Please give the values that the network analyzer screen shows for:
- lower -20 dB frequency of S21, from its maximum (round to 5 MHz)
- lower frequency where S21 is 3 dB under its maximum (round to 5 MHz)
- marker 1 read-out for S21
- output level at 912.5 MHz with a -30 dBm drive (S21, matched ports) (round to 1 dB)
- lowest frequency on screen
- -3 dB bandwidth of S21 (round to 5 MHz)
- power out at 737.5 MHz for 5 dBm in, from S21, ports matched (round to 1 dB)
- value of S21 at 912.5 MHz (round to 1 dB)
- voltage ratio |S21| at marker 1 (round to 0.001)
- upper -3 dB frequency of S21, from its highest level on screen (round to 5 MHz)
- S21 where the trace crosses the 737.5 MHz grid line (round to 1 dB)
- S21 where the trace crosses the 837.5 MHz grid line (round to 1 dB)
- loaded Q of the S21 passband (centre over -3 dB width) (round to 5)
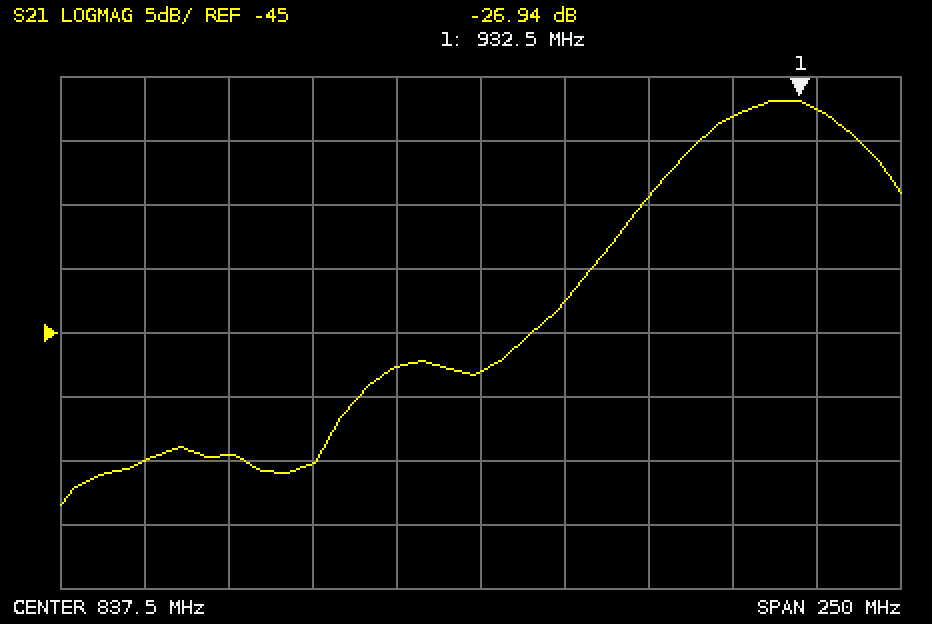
845 MHz
905 MHz
-26.94 dB
-58 dBm
712.5 MHz
45 MHz
-50 dBm
-28 dB
0.045
950 MHz
-55 dB
-48 dB
20
